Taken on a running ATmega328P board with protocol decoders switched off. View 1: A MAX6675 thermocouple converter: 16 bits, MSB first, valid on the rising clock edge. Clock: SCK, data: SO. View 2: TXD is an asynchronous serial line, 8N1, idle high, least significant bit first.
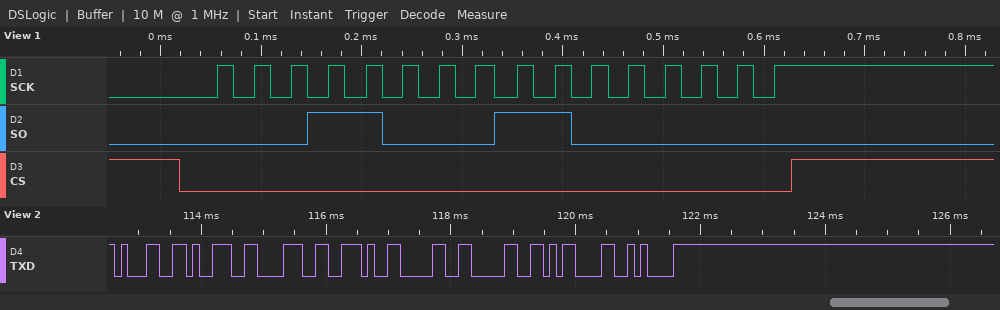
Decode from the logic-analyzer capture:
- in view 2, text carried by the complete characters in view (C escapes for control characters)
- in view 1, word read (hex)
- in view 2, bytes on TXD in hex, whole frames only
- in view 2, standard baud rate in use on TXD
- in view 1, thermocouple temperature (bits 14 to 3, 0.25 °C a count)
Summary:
"198.00\r\n"
0x18C0
31 39 38 2E 30 30 0D 0A
9600 baud
198.00 °C
